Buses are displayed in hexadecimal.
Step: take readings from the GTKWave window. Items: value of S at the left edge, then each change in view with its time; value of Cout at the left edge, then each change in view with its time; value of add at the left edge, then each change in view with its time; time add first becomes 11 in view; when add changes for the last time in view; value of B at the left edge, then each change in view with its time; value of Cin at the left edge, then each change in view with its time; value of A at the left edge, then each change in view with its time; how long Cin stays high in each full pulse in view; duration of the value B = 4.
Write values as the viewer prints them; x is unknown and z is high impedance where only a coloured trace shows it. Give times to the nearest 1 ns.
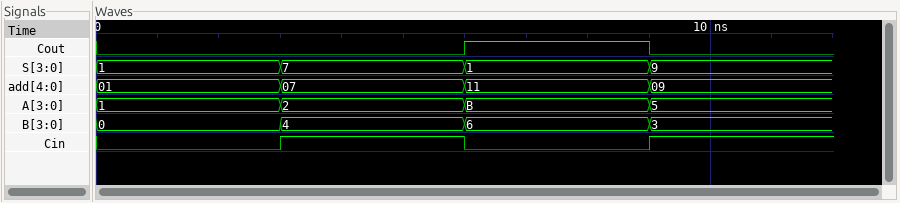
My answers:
1, 7 at 3 ns, 1 at 6 ns, 9 at 9 ns
0, 1 at 6 ns, 0 at 9 ns
01, 07 at 3 ns, 11 at 6 ns, 09 at 9 ns
6 ns
9 ns
0, 4 at 3 ns, 6 at 6 ns, 3 at 9 ns
0, 1 at 3 ns, 0 at 6 ns, 1 at 9 ns
1, 2 at 3 ns, B at 6 ns, 5 at 9 ns
3 ns
3 ns
